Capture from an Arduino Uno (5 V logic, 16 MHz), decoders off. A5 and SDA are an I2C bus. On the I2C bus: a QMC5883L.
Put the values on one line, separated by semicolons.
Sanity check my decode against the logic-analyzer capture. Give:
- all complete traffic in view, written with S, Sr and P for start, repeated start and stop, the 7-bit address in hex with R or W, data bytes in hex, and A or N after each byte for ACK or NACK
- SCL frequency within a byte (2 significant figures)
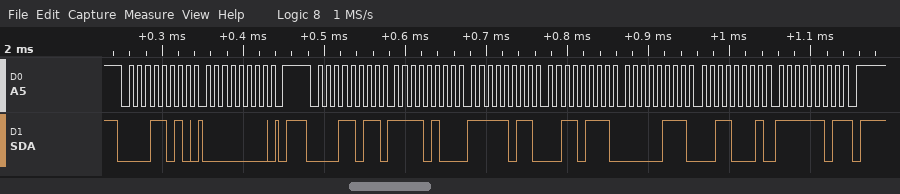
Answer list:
S 0DW A 00 A P S 0DR A F4 A FB A 37 A 07 A 31 A FD N P; 100 kHz
